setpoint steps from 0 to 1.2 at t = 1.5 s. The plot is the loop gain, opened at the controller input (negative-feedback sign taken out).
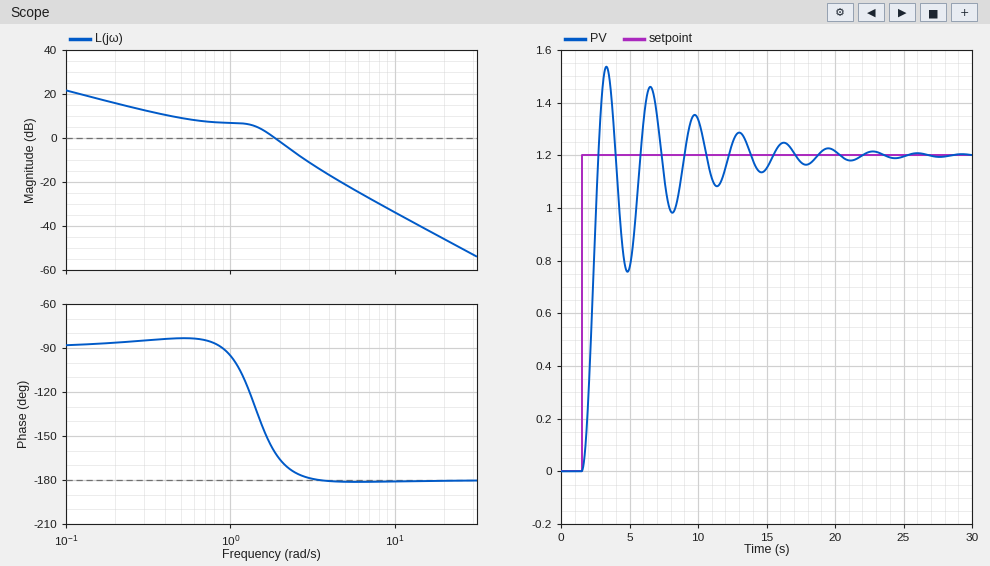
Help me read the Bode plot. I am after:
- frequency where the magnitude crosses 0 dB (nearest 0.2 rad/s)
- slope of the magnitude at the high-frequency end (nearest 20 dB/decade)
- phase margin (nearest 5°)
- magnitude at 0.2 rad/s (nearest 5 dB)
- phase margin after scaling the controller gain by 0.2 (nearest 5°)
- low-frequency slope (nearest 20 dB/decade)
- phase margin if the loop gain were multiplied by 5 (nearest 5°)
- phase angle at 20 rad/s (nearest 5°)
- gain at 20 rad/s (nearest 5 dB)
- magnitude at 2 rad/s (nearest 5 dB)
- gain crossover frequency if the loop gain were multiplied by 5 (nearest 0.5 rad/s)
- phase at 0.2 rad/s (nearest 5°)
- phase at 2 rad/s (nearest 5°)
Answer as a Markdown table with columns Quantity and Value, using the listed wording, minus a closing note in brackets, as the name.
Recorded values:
| Quantity | Value |
|---|---|
| frequency where the magnitude crosses 0 dB | 1.8 rad/s |
| slope of the magnitude at the high-frequency end | -40 dB/decade |
| phase margin | 20° |
| magnitude at 0.2 rad/s | 15 dB |
| phase margin after scaling the controller gain by 0.2 | 95° |
| low-frequency slope | -20 dB/decade |
| phase margin if the loop gain were multiplied by 5 | 0° |
| phase angle at 20 rad/s | -180° |
| gain at 20 rad/s | -45 dB |
| magnitude at 2 rad/s | 0 dB |
| gain crossover frequency if the loop gain were multiplied by 5 | 3.5 rad/s |
| phase at 0.2 rad/s | -85° |
| phase at 2 rad/s | -165° |
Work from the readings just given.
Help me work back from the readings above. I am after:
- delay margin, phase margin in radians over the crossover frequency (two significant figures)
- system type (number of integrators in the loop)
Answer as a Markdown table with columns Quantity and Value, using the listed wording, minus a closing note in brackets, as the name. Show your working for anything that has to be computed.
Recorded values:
| Quantity | Value |
|---|---|
| delay margin, phase margin in radians over the crossover frequency | 20 × π / 180 / 1.8 = 0.19 s |
| system type | 1 |
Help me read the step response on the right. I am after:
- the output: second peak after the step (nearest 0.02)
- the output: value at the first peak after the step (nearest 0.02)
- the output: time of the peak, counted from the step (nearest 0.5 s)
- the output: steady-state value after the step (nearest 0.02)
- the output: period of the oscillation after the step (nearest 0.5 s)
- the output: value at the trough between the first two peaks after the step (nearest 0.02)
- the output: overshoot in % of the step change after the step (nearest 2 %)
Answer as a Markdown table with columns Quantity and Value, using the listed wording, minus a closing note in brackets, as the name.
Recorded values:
| Quantity | Value |
|---|---|
| the output: second peak after the step | 1.46 |
| the output: value at the first peak after the step | 1.54 |
| the output: time of the peak, counted from the step | 2.0 s |
| the output: steady-state value after the step | 1.20 |
| the output: period of the oscillation after the step | 3.0 s |
| the output: value at the trough between the first two peaks after the step | 0.76 |
| the output: overshoot in % of the step change after the step | 28 % |
